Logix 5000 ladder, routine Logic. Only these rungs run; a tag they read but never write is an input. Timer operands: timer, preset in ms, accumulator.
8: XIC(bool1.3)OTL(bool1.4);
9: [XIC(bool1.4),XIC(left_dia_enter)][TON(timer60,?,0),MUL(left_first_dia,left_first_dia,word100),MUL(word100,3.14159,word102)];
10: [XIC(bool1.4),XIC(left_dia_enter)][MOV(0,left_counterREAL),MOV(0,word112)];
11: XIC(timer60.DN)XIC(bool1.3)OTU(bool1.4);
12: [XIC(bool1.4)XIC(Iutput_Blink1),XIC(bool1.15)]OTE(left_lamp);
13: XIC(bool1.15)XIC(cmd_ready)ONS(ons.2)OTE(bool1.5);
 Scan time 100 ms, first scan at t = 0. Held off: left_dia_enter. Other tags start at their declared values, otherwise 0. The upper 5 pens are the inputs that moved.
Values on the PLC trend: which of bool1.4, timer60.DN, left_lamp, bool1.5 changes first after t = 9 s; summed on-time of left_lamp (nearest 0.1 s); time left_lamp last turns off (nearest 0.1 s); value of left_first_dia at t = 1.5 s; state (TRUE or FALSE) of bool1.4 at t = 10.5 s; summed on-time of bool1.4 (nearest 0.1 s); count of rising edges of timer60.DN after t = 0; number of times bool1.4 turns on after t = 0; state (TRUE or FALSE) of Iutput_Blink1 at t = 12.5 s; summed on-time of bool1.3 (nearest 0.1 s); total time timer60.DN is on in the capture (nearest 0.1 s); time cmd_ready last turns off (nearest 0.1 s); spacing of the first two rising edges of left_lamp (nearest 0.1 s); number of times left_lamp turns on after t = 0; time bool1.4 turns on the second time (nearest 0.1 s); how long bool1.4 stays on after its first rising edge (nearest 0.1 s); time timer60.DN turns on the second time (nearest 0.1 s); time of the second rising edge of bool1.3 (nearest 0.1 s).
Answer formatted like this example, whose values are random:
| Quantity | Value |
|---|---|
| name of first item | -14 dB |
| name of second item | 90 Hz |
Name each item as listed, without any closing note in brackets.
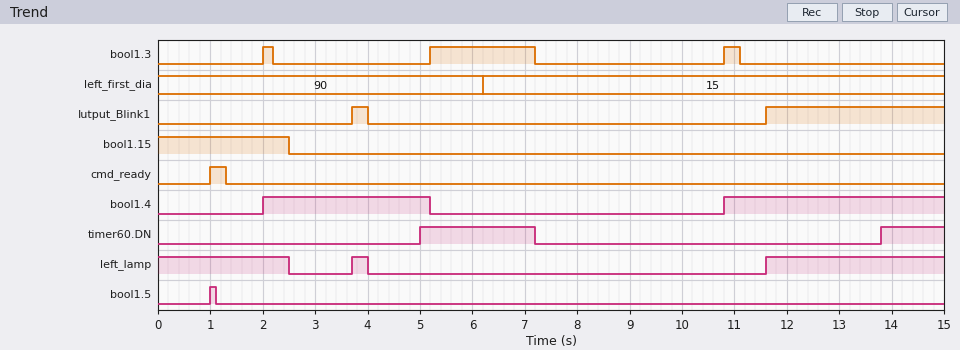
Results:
| Quantity | Value |
|---|---|
| which of bool1.4, timer60.DN, left_lamp, bool1.5 changes first after t = 9 s | bool1.4 |
| summed on-time of left_lamp | 6.2 s |
| time left_lamp last turns off | 4.0 s |
| value of left_first_dia at t = 1.5 s | 90 |
| state (TRUE or FALSE) of bool1.4 at t = 10.5 s | FALSE |
| summed on-time of bool1.4 | 7.4 s |
| count of rising edges of timer60.DN after t = 0 | 2 |
| number of times bool1.4 turns on after t = 0 | 2 |
| state (TRUE or FALSE) of Iutput_Blink1 at t = 12.5 s | TRUE |
| summed on-time of bool1.3 | 2.5 s |
| total time timer60.DN is on in the capture | 3.4 s |
| time cmd_ready last turns off | 1.3 s |
| spacing of the first two rising edges of left_lamp | 7.9 s |
| number of times left_lamp turns on after t = 0 | 2 |
| time bool1.4 turns on the second time | 10.8 s |
| how long bool1.4 stays on after its first rising edge | 3.2 s |
| time timer60.DN turns on the second time | 13.8 s |
| time of the second rising edge of bool1.3 | 5.2 s |
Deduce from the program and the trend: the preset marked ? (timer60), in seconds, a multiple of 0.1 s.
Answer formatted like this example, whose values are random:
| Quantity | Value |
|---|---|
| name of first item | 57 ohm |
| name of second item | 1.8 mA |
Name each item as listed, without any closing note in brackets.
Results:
| Quantity | Value |
|---|---|
| the preset marked ? (timer60), in seconds, a multiple of 0.1 s | 3.0 s |
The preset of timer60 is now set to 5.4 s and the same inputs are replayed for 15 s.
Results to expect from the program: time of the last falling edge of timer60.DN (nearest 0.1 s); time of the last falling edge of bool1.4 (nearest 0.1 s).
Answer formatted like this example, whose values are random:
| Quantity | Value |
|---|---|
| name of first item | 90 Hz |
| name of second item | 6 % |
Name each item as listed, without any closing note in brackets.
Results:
| Quantity | Value |
|---|---|
| time of the last falling edge of timer60.DN | 11.1 s |
| time of the last falling edge of bool1.4 | 10.8 s |
